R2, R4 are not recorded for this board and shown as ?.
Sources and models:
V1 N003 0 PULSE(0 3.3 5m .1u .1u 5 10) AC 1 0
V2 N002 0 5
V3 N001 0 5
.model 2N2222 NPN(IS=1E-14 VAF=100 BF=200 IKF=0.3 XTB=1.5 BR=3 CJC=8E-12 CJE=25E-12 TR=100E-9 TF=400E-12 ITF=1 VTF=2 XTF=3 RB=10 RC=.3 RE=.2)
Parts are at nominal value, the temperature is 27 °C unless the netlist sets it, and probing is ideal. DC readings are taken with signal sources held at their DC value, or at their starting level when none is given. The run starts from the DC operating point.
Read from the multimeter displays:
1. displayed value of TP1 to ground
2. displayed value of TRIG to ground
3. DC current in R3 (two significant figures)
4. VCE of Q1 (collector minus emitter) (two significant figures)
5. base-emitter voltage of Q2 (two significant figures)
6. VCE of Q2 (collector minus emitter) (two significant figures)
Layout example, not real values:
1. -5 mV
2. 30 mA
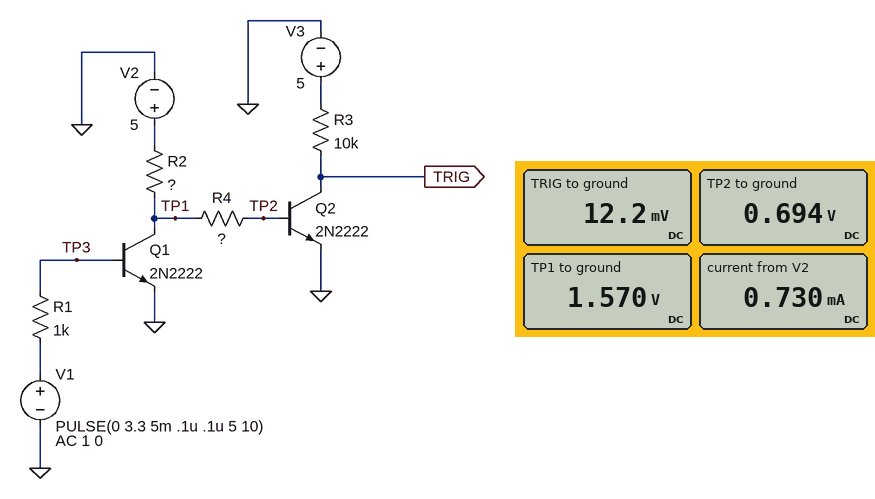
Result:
1. 1.570 V
2. 12.2 mV
3. 500 µA
4. 1.6 V
5. 690 mV
6. 12 mV
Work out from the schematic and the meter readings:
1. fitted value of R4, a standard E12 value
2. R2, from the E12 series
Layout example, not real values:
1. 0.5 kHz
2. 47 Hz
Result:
1. 1.2 kΩ
2. 4.7 kΩ
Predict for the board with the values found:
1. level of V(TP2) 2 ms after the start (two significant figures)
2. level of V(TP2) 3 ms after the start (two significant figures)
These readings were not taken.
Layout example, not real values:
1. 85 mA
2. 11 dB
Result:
1. 690 mV
2. 690 mV
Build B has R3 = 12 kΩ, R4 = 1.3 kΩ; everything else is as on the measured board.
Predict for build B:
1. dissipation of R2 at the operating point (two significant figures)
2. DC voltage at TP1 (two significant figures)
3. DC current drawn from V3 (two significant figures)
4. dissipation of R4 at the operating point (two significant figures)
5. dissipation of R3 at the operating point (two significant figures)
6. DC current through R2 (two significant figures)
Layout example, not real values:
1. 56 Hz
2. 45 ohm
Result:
1. 2.4 mW
2. 1.6 V
3. 420 µA
4. 670 µW
5. 2.1 mW
6. 720 µA
